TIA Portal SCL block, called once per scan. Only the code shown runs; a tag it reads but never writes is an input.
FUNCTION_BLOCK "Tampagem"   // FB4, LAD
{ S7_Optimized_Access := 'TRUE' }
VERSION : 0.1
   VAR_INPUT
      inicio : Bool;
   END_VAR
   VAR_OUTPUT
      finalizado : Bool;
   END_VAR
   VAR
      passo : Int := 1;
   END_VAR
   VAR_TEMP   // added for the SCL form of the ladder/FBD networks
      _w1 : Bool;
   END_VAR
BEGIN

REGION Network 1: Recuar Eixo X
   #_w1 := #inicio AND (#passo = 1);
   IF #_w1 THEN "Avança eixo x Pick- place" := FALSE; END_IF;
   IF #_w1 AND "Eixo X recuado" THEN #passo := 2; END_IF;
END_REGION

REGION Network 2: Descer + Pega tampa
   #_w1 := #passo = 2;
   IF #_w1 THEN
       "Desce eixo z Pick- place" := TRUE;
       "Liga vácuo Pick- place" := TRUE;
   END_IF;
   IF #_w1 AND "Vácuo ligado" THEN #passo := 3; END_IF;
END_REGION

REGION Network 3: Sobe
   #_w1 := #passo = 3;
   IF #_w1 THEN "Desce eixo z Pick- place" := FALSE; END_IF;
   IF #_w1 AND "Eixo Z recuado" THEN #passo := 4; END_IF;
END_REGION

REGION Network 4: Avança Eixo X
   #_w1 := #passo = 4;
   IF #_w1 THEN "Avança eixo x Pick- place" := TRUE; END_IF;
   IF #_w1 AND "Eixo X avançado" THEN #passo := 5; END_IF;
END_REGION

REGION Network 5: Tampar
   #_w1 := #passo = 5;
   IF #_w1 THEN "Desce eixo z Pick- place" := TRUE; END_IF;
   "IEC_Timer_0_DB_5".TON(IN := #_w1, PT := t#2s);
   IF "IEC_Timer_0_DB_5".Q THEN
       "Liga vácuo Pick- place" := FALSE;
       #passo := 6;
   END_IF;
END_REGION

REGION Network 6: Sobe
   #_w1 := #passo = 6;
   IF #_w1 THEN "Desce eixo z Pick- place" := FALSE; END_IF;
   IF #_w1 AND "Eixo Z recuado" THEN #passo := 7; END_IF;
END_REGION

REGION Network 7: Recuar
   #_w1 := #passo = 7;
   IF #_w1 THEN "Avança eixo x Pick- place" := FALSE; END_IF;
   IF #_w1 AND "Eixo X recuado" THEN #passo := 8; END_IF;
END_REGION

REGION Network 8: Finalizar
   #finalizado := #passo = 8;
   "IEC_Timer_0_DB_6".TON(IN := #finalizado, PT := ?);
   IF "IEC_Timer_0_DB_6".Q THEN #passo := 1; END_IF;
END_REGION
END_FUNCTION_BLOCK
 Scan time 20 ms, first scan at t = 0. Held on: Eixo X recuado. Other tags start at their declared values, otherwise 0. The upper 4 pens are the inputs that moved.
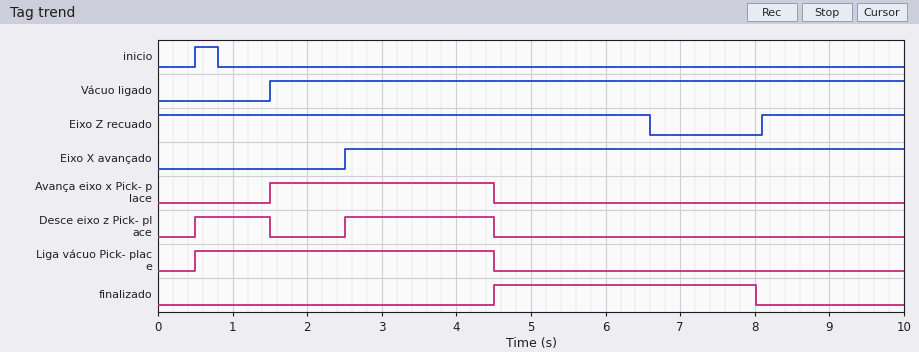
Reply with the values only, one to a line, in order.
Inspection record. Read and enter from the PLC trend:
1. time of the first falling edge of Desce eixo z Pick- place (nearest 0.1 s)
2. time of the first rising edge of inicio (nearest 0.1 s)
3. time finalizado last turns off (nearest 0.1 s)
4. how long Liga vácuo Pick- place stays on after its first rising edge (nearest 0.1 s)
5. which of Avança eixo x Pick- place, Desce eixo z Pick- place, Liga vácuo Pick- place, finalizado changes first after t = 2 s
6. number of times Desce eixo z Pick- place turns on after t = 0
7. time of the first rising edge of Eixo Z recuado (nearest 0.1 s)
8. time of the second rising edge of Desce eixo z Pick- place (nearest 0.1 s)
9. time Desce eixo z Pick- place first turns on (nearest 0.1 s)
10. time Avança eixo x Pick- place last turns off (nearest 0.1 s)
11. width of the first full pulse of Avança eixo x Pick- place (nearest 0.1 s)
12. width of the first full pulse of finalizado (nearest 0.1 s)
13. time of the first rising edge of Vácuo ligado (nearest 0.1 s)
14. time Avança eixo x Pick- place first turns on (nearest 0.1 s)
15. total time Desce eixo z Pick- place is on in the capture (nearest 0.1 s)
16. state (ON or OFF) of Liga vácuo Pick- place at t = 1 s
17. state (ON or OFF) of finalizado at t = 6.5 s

1.5 s
0.5 s
8.0 s
4.0 s
Desce eixo z Pick- place
2
8.1 s
2.5 s
0.5 s
4.5 s
3.0 s
3.5 s
1.5 s
1.5 s
3.0 s
ON
ON
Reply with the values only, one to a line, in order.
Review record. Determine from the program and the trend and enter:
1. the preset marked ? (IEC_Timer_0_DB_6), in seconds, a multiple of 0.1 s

3.5 s
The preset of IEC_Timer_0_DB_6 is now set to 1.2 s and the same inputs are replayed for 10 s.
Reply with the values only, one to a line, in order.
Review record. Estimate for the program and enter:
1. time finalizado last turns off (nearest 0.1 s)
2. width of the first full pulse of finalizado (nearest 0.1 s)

5.7 s
1.2 s
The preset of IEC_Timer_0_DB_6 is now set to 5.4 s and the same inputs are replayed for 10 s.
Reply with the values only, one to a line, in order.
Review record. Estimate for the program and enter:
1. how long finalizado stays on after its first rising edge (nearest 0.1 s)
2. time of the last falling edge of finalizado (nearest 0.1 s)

5.4 s
9.9 s
